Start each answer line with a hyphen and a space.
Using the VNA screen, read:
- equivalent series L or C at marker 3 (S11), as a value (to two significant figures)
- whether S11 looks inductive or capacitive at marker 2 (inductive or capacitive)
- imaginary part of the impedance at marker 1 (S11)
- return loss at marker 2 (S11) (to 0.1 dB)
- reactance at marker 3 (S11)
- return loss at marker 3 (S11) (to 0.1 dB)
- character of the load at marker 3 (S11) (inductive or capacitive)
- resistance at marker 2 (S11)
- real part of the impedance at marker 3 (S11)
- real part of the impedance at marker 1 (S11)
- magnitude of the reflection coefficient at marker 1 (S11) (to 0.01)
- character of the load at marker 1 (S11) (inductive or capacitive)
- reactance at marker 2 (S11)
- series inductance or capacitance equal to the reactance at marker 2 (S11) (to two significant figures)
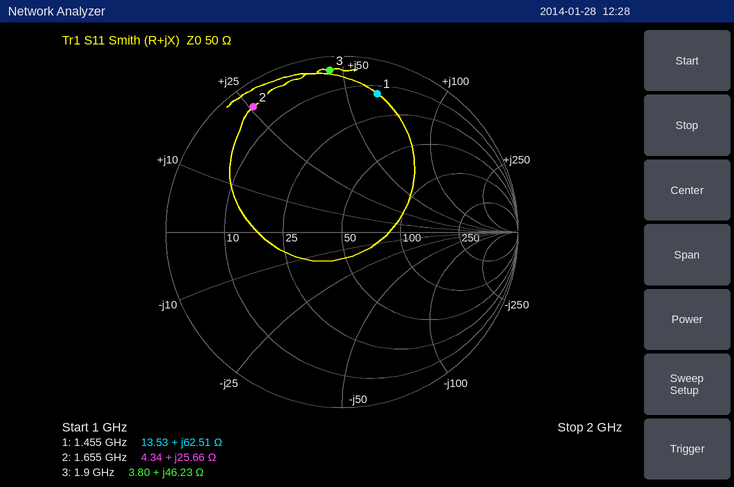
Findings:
- 3.9 nH
- inductive
- +62.51 Ω
- 1.2 dB
- +46.23 Ω
- 0.7 dB
- inductive
- 4.34 Ω
- 3.80 Ω
- 13.53 Ω
- 0.81
- inductive
- +25.66 Ω
- 2.5 nH
